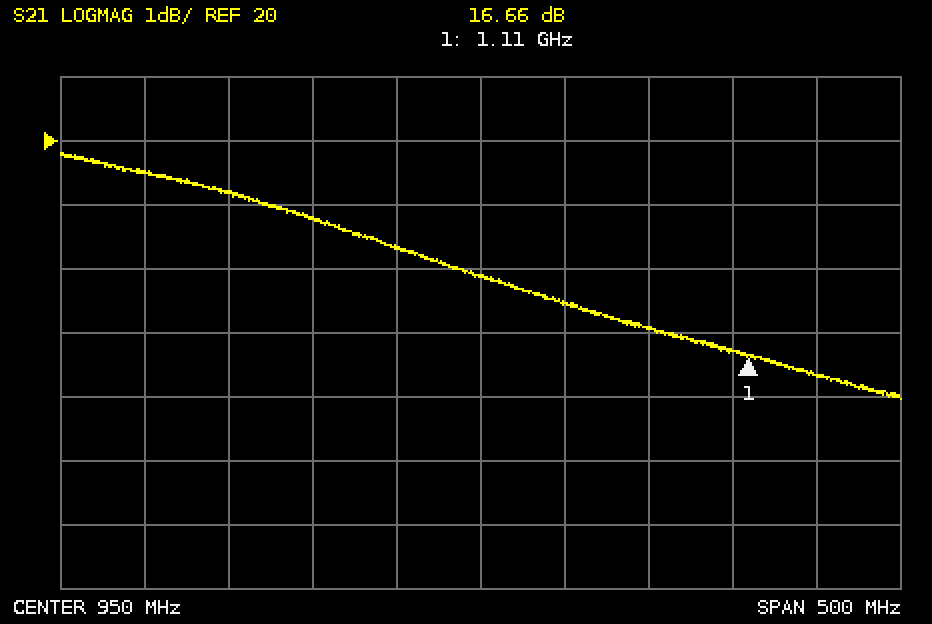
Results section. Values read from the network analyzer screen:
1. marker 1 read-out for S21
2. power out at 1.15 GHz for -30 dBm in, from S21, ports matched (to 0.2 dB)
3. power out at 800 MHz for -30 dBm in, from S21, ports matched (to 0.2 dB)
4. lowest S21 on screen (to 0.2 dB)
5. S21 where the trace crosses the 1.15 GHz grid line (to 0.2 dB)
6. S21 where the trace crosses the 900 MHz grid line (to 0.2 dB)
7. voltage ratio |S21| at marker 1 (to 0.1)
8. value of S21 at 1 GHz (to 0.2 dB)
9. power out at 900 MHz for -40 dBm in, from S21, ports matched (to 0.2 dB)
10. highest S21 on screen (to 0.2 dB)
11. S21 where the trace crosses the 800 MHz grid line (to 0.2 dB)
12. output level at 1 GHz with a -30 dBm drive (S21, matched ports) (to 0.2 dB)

16.66 dB
-13.6 dBm
-10.8 dBm
16.0 dB
16.4 dB
18.4 dB
6.8
17.4 dB
-21.6 dBm
19.8 dB
19.2 dB
-12.6 dBm
